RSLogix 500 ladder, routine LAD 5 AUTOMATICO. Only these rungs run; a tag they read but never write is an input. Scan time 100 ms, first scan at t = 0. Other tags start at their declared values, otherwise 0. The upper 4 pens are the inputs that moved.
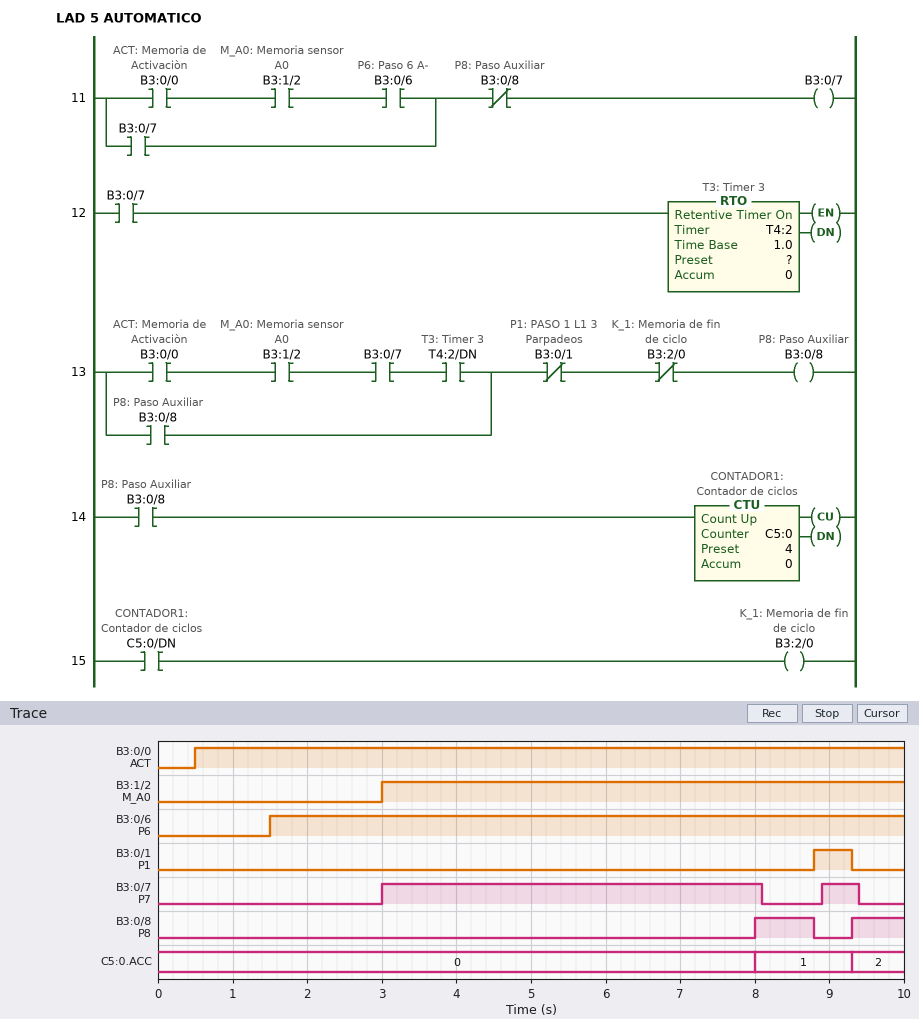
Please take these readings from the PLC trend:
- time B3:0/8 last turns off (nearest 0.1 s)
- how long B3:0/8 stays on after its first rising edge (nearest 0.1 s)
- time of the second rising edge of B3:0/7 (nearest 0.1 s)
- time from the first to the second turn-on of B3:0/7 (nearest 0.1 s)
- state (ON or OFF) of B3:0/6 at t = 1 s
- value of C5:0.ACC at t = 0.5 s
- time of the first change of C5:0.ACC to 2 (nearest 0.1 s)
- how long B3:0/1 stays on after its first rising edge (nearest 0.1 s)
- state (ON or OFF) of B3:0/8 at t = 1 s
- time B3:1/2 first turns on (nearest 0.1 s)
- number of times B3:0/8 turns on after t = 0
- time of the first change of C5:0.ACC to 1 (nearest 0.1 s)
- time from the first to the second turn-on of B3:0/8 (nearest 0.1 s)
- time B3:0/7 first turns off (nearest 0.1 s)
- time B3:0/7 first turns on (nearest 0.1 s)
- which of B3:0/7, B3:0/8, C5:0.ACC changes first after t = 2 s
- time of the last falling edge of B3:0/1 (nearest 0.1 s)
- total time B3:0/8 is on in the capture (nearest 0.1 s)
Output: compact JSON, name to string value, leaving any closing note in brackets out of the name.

{"time B3:0/8 last turns off": "8.8 s", "how long B3:0/8 stays on after its first rising edge": "0.8 s", "time of the second rising edge of B3:0/7": "8.9 s", "time from the first to the second turn-on of B3:0/7": "5.9 s", "state (ON or OFF) of B3:0/6 at t = 1 s": "OFF", "value of C5:0.ACC at t = 0.5 s": "0", "time of the first change of C5:0.ACC to 2": "9.3 s", "how long B3:0/1 stays on after its first rising edge": "0.5 s", "state (ON or OFF) of B3:0/8 at t = 1 s": "OFF", "time B3:1/2 first turns on": "3.0 s", "number of times B3:0/8 turns on after t = 0": "2", "time of the first change of C5:0.ACC to 1": "8.0 s", "time from the first to the second turn-on of B3:0/8": "1.3 s", "time B3:0/7 first turns off": "8.1 s", "time B3:0/7 first turns on": "3.0 s", "which of B3:0/7, B3:0/8, C5:0.ACC changes first after t = 2 s": "B3:0/7", "time of the last falling edge of B3:0/1": "9.3 s", "total time B3:0/8 is on in the capture": "1.5 s"}
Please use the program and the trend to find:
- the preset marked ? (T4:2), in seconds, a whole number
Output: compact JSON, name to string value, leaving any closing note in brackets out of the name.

{"the preset marked ? (T4:2), in seconds, a whole number": "5 s"}
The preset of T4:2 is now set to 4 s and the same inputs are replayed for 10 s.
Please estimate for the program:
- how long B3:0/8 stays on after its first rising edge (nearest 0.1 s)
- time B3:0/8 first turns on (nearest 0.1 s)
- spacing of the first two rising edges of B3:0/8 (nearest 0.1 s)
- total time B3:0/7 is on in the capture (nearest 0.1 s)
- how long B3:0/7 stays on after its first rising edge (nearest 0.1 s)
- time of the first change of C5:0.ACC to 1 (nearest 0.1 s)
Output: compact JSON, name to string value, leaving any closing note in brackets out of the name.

{"how long B3:0/8 stays on after its first rising edge": "1.8 s", "time B3:0/8 first turns on": "7.0 s", "spacing of the first two rising edges of B3:0/8": "2.3 s", "total time B3:0/7 is on in the capture": "4.6 s", "how long B3:0/7 stays on after its first rising edge": "4.1 s", "time of the first change of C5:0.ACC to 1": "7.0 s"}
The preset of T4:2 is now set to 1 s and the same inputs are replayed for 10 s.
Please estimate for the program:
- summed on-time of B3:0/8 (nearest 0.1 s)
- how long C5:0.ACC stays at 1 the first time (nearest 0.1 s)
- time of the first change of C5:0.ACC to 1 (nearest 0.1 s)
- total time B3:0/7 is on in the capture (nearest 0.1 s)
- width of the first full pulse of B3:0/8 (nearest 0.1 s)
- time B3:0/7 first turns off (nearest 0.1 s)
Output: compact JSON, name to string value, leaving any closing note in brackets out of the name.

{"summed on-time of B3:0/8": "5.5 s", "how long C5:0.ACC stays at 1 the first time": "5.3 s", "time of the first change of C5:0.ACC to 1": "4.0 s", "total time B3:0/7 is on in the capture": "1.6 s", "width of the first full pulse of B3:0/8": "4.8 s", "time B3:0/7 first turns off": "4.1 s"}
